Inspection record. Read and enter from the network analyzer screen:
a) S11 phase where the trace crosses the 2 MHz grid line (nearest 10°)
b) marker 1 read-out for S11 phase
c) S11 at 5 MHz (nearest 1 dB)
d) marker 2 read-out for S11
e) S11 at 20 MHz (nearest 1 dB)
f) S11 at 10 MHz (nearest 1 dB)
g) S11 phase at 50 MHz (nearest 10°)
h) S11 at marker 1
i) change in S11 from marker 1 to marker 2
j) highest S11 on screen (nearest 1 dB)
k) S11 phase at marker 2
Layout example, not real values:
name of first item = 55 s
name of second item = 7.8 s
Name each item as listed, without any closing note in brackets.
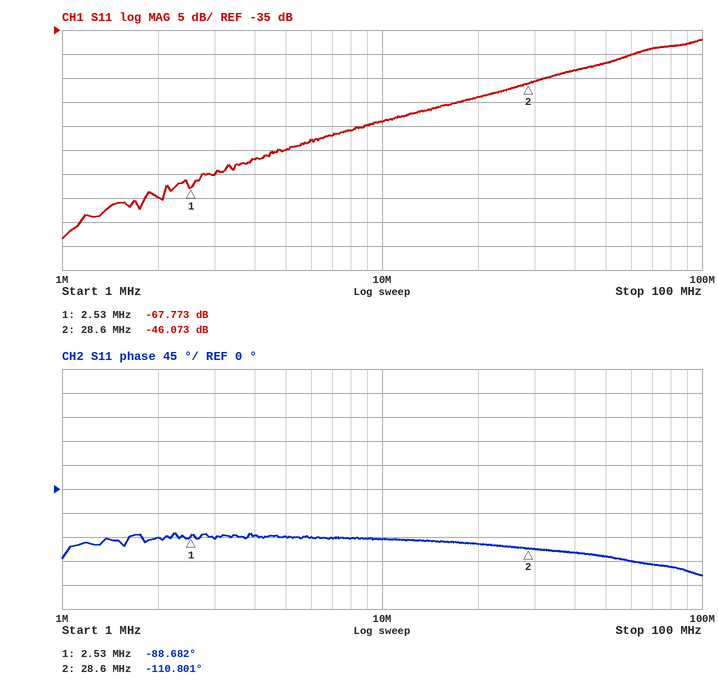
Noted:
S11 phase where the trace crosses the 2 MHz grid line = -90°
marker 1 read-out for S11 phase = -88.682°
S11 at 5 MHz = -60 dB
marker 2 read-out for S11 = -46.073 dB
S11 at 20 MHz = -49 dB
S11 at 10 MHz = -54 dB
S11 phase at 50 MHz = -130°
S11 at marker 1 = -67.773 dB
change in S11 from marker 1 to marker 2 = 21.700 dB
highest S11 on screen = -37 dB
S11 phase at marker 2 = -110.801°
